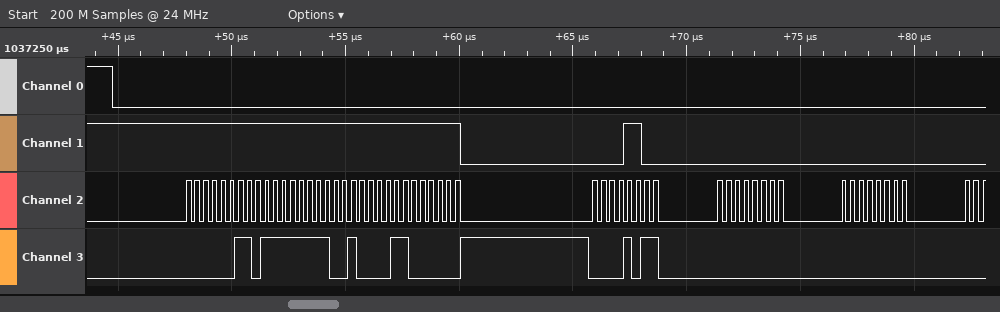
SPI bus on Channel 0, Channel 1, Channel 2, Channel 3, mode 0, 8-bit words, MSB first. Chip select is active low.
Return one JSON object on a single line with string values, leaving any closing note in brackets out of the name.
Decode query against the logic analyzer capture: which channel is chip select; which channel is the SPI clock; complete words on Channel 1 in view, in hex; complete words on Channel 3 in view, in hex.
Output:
{"which channel is chip select": "Channel 0", "which channel is the SPI clock": "Channel 2", "complete words on Channel 1 in view, in hex": "FF, FF, FF, FF, 0C, 00, 00", "complete words on Channel 3 in view, in hex": "03, 7F, 90, C0, 0B, 00, 00"}
